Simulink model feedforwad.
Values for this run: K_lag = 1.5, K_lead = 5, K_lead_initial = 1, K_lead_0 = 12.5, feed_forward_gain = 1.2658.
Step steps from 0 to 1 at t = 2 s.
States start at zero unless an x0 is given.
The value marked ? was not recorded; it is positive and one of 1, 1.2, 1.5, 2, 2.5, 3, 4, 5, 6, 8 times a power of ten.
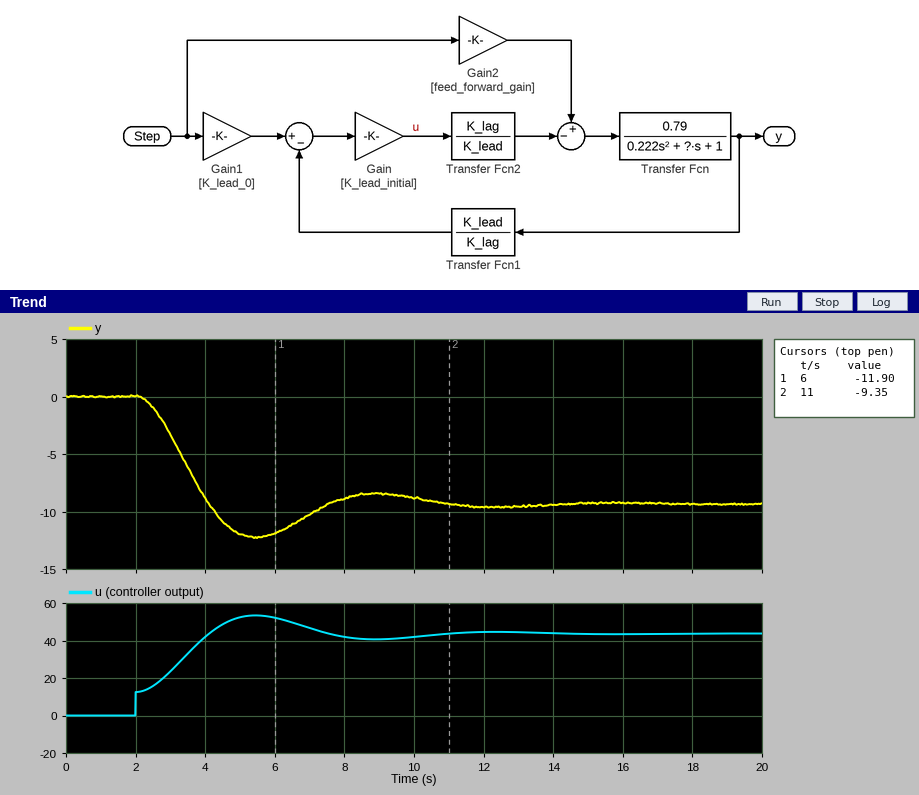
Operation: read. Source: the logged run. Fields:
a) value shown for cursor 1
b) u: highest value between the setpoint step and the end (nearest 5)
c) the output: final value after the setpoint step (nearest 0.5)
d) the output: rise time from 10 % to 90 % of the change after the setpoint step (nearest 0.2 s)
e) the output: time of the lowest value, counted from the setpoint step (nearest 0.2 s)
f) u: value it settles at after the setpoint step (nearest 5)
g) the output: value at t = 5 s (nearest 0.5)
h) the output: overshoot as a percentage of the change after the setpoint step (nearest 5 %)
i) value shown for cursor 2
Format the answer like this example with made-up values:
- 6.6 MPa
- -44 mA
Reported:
- -11.90
- 55
- -9.5
- 1.4 s
- 3.4 s
- 45
- -12.0
- 30 %
- -9.35
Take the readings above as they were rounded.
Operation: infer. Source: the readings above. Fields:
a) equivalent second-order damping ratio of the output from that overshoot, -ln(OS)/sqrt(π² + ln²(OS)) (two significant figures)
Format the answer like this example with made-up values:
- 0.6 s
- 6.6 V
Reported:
- 0.36
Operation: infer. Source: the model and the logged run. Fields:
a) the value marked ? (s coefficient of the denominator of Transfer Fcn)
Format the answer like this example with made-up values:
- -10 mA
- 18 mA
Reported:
- 0.15
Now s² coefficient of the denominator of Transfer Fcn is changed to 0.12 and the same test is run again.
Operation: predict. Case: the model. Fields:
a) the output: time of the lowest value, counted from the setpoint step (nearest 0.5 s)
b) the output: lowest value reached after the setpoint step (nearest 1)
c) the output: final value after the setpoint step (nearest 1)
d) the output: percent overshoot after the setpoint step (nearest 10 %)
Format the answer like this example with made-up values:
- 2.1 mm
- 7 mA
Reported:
- 2.5 s
- -11
- -9
- 20 %
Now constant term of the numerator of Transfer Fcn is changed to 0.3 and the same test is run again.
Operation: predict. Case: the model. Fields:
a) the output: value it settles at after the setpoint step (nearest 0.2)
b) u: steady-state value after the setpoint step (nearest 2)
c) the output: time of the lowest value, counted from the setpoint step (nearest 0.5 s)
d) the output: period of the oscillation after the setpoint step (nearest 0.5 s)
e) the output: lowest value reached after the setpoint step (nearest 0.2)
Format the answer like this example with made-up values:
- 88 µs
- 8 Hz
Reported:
- -1.0
- 16
- 2.0 s
- 3.5 s
- -1.6
